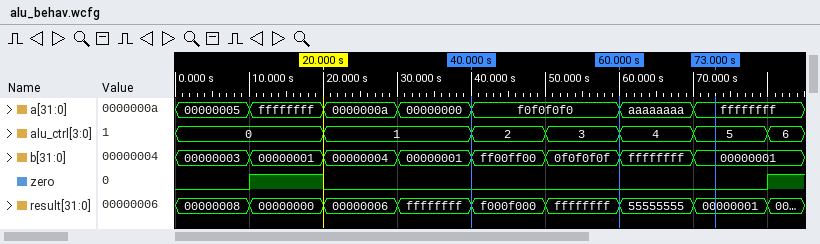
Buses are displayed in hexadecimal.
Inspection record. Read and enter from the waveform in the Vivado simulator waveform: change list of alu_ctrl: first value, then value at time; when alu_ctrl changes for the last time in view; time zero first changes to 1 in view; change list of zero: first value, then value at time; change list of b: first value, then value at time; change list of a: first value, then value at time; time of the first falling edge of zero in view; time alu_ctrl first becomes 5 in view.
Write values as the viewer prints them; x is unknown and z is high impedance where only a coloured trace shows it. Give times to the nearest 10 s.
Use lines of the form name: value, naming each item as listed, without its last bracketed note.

change list of alu_ctrl: first value, then value at time: 0, 1 at 20 s, 2 at 40 s, 3 at 50 s, 4 at 60 s, 5 at 70 s, 6 at 80 s
when alu_ctrl changes for the last time in view: 80 s
time zero first changes to 1 in view: 10 s
change list of zero: first value, then value at time: 0, 1 at 10 s, 0 at 20 s, 1 at 80 s
change list of b: first value, then value at time: 00000003, 00000001 at 10 s, 00000004 at 20 s, 00000001 at 30 s, ff00ff00 at 40 s, 0f0f0f0f at 50 s, ffffffff at 60 s, 00000001 at 70 s
change list of a: first value, then value at time: 00000005, ffffffff at 10 s, 0000000a at 20 s, 00000000 at 30 s, f0f0f0f0 at 40 s, aaaaaaaa at 60 s, ffffffff at 70 s
time of the first falling edge of zero in view: 20 s
time alu_ctrl first becomes 5 in view: 70 s
